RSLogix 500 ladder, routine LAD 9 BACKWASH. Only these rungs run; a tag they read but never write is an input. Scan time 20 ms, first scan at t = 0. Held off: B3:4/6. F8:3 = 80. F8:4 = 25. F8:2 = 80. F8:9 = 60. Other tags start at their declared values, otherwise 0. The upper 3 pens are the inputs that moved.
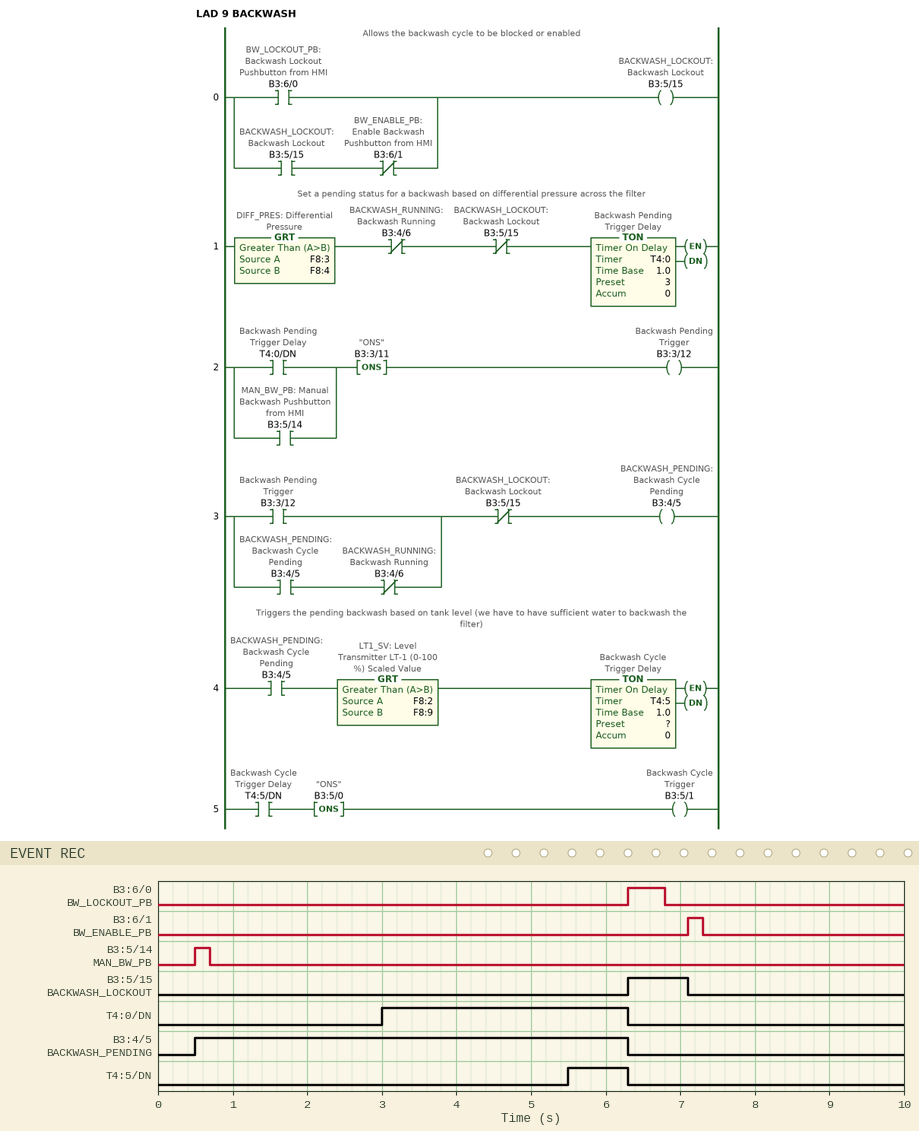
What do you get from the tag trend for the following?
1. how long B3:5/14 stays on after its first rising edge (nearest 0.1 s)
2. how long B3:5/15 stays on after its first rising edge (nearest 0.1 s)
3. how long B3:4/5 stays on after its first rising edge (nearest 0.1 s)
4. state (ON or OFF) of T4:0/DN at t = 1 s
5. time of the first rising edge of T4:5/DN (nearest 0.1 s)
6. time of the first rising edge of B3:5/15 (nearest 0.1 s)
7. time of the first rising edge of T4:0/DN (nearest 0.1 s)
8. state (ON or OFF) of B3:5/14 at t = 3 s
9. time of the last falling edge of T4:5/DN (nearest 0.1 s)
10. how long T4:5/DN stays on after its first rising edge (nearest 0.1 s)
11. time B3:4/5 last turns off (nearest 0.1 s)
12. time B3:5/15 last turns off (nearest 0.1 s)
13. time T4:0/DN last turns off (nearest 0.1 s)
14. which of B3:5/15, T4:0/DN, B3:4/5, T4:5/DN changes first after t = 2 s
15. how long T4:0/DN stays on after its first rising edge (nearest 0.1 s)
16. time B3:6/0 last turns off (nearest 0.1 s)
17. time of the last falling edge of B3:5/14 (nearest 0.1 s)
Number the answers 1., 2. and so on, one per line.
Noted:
1. 0.2 s
2. 0.8 s
3. 5.8 s
4. OFF
5. 5.5 s
6. 6.3 s
7. 3.0 s
8. OFF
9. 6.3 s
10. 0.8 s
11. 6.3 s
12. 7.1 s
13. 6.3 s
14. T4:0/DN
15. 3.3 s
16. 6.8 s
17. 0.7 s
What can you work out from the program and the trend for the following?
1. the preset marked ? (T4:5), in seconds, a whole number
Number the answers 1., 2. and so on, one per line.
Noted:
1. 5 s
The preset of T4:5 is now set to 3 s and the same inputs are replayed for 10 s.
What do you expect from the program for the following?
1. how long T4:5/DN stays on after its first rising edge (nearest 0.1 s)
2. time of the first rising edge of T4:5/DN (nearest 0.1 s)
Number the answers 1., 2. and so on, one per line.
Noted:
1. 2.8 s
2. 3.5 s
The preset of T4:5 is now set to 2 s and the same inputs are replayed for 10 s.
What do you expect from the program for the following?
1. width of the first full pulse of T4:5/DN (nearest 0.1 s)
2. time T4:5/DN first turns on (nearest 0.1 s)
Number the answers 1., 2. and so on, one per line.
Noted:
1. 3.8 s
2. 2.5 s
